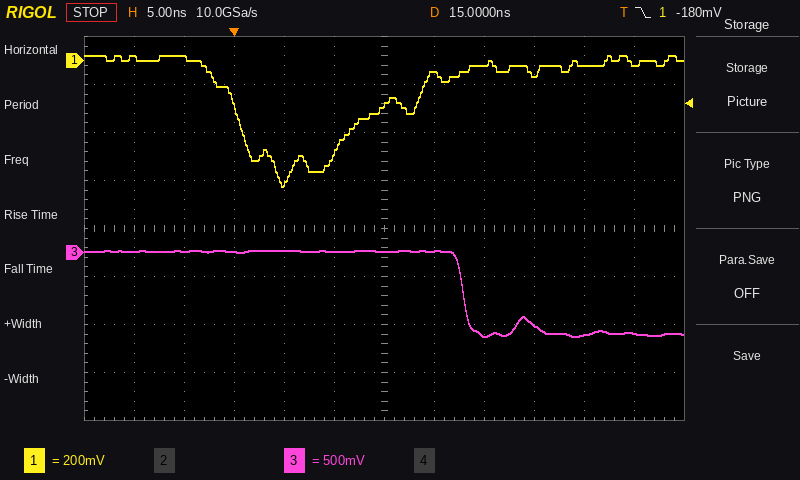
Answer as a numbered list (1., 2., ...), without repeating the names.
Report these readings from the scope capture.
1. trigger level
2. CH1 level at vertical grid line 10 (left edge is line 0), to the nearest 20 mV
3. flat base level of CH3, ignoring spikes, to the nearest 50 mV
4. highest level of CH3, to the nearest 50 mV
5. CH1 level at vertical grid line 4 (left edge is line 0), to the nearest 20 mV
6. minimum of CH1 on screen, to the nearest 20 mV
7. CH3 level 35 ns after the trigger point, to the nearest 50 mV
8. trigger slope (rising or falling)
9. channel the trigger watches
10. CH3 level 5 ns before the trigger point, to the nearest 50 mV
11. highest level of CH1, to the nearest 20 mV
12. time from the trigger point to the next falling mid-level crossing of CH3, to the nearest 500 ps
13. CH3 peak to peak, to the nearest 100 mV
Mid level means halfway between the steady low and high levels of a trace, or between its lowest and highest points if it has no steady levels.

1. -180 mV
2. -20 mV
3. -850 mV
4. 0 mV
5. -520 mV
6. -520 mV
7. -850 mV
8. falling
9. CH1
10. 0 mV
11. 20 mV
12. 23.0 ns
13. 900 mV
